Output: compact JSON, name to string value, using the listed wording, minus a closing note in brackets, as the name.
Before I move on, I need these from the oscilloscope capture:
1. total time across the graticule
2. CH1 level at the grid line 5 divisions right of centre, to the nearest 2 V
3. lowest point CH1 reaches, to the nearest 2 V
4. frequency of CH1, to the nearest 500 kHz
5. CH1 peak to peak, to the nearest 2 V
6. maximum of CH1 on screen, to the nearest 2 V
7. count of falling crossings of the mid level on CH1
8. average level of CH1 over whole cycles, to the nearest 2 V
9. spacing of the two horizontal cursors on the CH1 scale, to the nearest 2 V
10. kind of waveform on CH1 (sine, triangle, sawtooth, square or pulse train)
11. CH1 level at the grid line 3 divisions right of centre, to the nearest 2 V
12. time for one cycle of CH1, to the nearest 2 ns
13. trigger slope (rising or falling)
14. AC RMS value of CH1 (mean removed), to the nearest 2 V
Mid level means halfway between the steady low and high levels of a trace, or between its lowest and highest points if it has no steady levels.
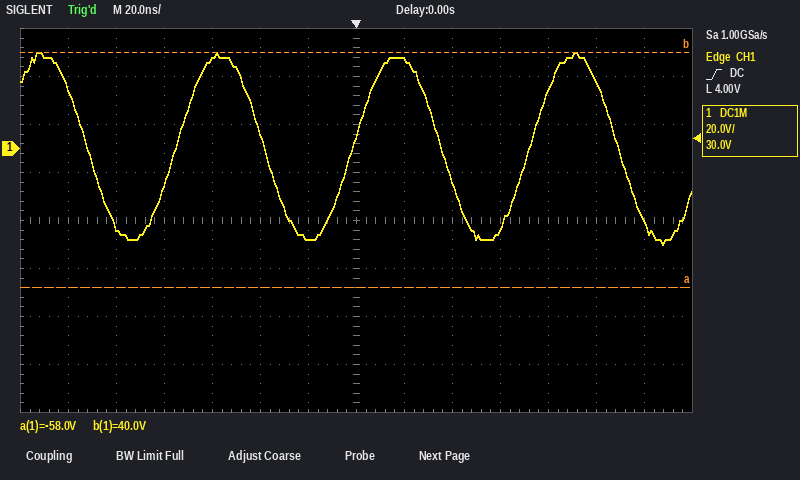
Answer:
{"total time across the graticule": "280 ns", "CH1 level at the grid line 5 divisions right of centre, to the nearest 2 V": "28 V", "lowest point CH1 reaches, to the nearest 2 V": "-40 V", "frequency of CH1, to the nearest 500 kHz": "13.5 MHz", "CH1 peak to peak, to the nearest 2 V": "80 V", "maximum of CH1 on screen, to the nearest 2 V": "40 V", "count of falling crossings of the mid level on CH1": "4", "average level of CH1 over whole cycles, to the nearest 2 V": "0 V", "spacing of the two horizontal cursors on the CH1 scale, to the nearest 2 V": "98 V", "kind of waveform on CH1": "sine", "CH1 level at the grid line 3 divisions right of centre, to the nearest 2 V": "-34 V", "time for one cycle of CH1, to the nearest 2 ns": "74 ns", "trigger slope": "rising", "AC RMS value of CH1 (mean removed), to the nearest 2 V": "28 V"}
